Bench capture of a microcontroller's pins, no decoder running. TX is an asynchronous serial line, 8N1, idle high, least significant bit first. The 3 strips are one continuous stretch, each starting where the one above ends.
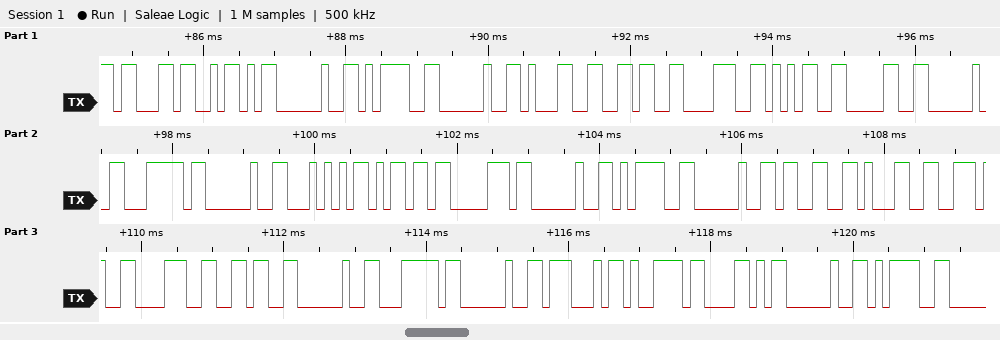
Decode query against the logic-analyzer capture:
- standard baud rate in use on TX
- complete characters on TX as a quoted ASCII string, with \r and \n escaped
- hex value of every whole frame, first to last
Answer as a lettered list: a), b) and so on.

a) 9600 baud
b) "cZ = 16850 | Tmp = 31.86 | GyX ="
c) 63 5A 20 3D 20 31 36 38 35 30 20 7C 20 54 6D 70 20 3D 20 33 31 2E 38 36 20 7C 20 47 79 58 20 3D
